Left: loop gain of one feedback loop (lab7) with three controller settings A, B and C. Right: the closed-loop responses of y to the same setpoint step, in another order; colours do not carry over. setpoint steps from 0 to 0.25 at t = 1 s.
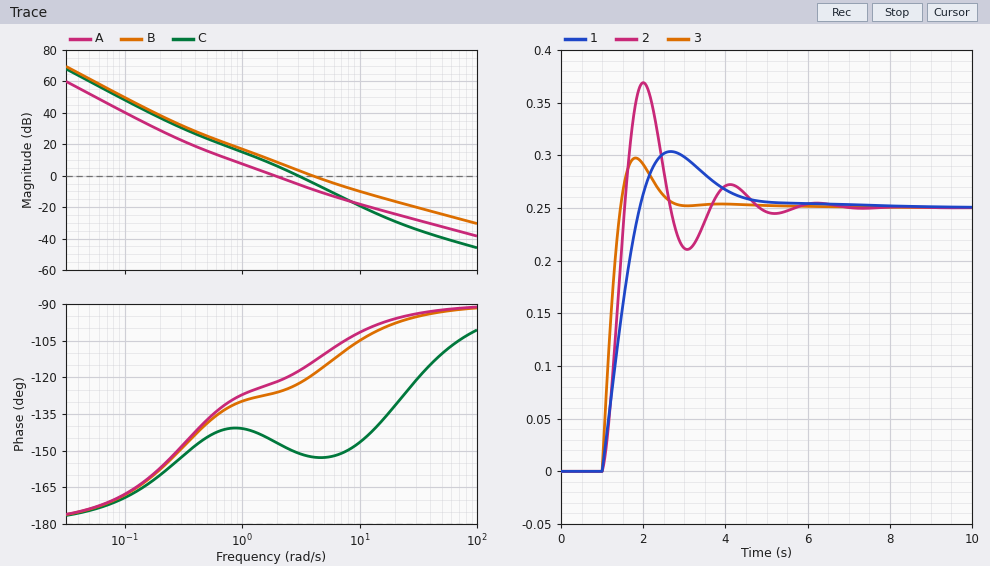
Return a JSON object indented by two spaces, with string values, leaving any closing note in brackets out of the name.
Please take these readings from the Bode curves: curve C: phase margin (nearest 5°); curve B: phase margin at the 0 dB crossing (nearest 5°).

{
  "curve C: phase margin": "30°",
  "curve B: phase margin at the 0 dB crossing": "60°"
}
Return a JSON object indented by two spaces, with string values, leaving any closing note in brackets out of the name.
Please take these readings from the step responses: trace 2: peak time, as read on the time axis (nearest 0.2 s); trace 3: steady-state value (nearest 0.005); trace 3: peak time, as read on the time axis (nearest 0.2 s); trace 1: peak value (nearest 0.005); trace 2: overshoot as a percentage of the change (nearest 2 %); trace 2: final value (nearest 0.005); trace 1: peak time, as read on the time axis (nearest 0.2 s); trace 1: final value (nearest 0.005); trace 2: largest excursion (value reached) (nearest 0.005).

{
  "trace 2: peak time, as read on the time axis": "2.0 s",
  "trace 3: steady-state value": "0.250",
  "trace 3: peak time, as read on the time axis": "1.8 s",
  "trace 1: peak value": "0.305",
  "trace 2: overshoot as a percentage of the change": "48 %",
  "trace 2: final value": "0.250",
  "trace 1: peak time, as read on the time axis": "2.6 s",
  "trace 1: final value": "0.250",
  "trace 2: largest excursion (value reached)": "0.370"
}
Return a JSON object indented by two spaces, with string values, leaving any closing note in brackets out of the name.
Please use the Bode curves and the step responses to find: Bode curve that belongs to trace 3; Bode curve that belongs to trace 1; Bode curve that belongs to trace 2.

{
  "Bode curve that belongs to trace 3": "B",
  "Bode curve that belongs to trace 1": "A",
  "Bode curve that belongs to trace 2": "C"
}
